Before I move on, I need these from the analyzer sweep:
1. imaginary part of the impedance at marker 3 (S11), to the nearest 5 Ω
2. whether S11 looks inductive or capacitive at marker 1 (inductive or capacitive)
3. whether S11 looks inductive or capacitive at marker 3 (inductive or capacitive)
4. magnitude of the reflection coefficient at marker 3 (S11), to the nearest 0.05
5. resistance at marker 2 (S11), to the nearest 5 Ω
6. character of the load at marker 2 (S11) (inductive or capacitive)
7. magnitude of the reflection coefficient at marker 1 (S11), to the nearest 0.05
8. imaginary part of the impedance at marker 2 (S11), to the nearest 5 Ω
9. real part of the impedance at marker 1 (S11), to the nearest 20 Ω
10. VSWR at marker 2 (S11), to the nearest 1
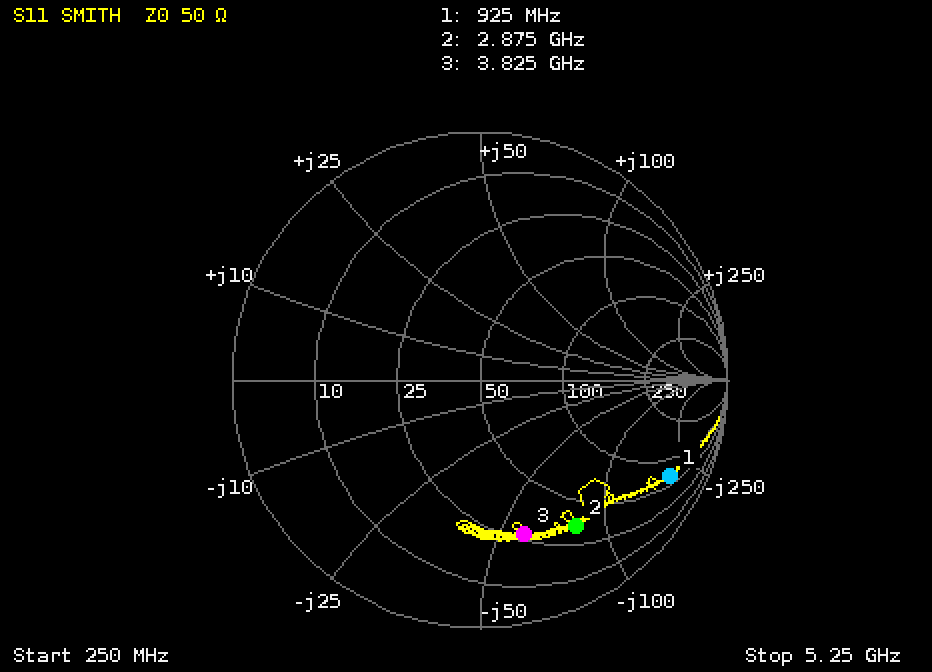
-60 Ω
capacitive
capacitive
0.65
35 Ω
capacitive
0.85
-80 Ω
60 Ω
6
